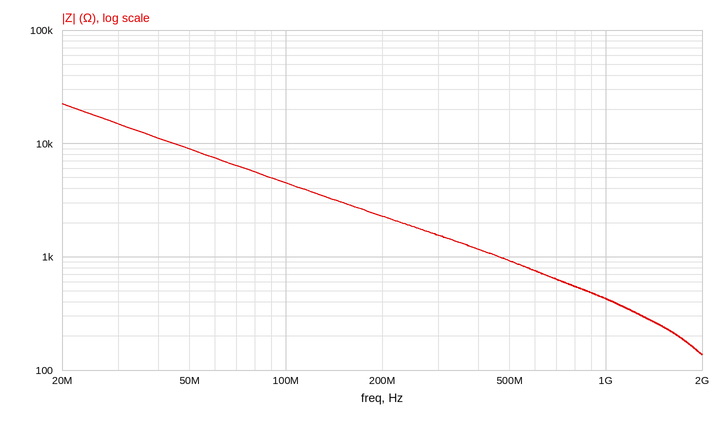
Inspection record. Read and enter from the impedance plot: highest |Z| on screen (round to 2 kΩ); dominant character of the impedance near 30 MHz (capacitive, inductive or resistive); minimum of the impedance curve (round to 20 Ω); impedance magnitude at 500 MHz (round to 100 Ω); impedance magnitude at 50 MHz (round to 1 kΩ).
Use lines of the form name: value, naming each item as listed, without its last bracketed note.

highest |Z| on screen: 22 kΩ
dominant character of the impedance near 30 MHz: capacitive
minimum of the impedance curve: 140 Ω
impedance magnitude at 500 MHz: 900 Ω
impedance magnitude at 50 MHz: 9 kΩ
